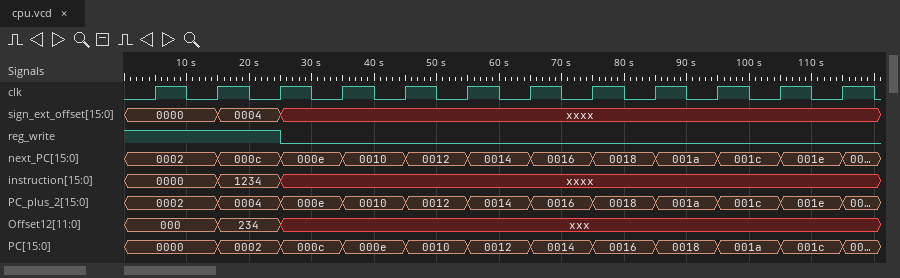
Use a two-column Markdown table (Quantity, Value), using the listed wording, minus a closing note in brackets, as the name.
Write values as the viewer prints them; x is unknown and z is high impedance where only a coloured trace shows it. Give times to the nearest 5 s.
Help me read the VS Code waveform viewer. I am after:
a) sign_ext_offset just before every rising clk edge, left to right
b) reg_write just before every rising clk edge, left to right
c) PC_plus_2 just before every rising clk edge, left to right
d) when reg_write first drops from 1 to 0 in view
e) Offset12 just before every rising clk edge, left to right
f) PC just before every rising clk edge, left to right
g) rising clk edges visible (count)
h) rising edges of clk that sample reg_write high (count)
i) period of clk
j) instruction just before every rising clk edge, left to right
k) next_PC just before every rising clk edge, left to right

| Quantity | Value |
|---|---|
| sign_ext_offset just before every rising clk edge, left to right | 0000, 0000, 0004, xxxx, xxxx, xxxx, xxxx, xxxx, xxxx, xxxx, xxxx, xxxx |
| reg_write just before every rising clk edge, left to right | 1 1 1 0 0 0 0 0 0 0 0 0 |
| PC_plus_2 just before every rising clk edge, left to right | 0002, 0002, 0004, 000e, 0010, 0012, 0014, 0016, 0018, 001a, 001c, 001e |
| when reg_write first drops from 1 to 0 in view | 25 s |
| Offset12 just before every rising clk edge, left to right | 000, 000, 234, xxx, xxx, xxx, xxx, xxx, xxx, xxx, xxx, xxx |
| PC just before every rising clk edge, left to right | 0000, 0000, 0002, 000c, 000e, 0010, 0012, 0014, 0016, 0018, 001a, 001c |
| rising clk edges visible | 12 |
| rising edges of clk that sample reg_write high | 3 |
| period of clk | 10 s |
| instruction just before every rising clk edge, left to right | 0000, 0000, 1234, xxxx, xxxx, xxxx, xxxx, xxxx, xxxx, xxxx, xxxx, xxxx |
| next_PC just before every rising clk edge, left to right | 0002, 0002, 000c, 000e, 0010, 0012, 0014, 0016, 0018, 001a, 001c, 001e |
